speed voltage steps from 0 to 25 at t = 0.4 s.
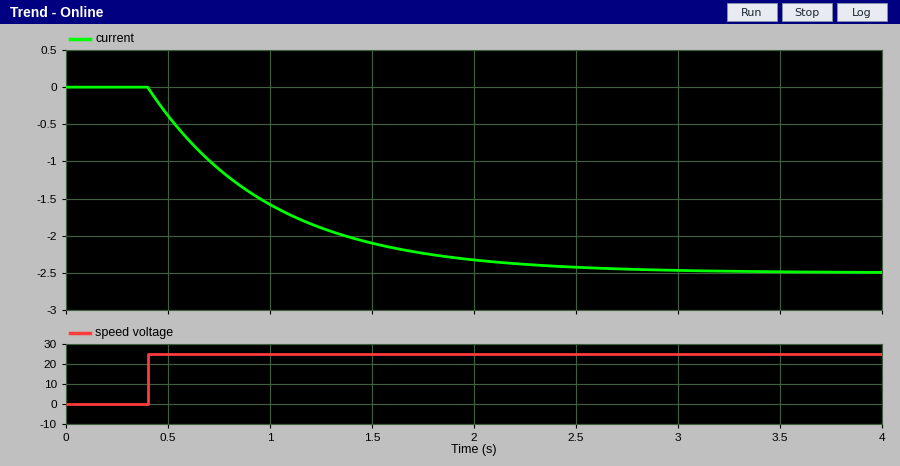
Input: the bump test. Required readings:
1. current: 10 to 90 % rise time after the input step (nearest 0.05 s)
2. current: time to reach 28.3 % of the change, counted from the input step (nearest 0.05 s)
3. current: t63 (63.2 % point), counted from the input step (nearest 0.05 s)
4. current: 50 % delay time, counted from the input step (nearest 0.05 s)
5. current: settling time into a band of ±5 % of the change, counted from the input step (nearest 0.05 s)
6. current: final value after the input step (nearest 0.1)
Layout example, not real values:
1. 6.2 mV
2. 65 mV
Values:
1. 1.30 s
2. 0.20 s
3. 0.60 s
4. 0.40 s
5. 1.80 s
6. -2.5
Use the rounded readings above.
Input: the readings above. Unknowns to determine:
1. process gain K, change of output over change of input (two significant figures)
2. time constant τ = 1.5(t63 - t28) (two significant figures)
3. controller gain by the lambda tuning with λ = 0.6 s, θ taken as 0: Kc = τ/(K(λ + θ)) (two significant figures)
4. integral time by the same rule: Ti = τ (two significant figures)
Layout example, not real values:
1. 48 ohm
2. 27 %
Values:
1. -0.10
2. 0.60 s
3. -10
4. 0.60 s
